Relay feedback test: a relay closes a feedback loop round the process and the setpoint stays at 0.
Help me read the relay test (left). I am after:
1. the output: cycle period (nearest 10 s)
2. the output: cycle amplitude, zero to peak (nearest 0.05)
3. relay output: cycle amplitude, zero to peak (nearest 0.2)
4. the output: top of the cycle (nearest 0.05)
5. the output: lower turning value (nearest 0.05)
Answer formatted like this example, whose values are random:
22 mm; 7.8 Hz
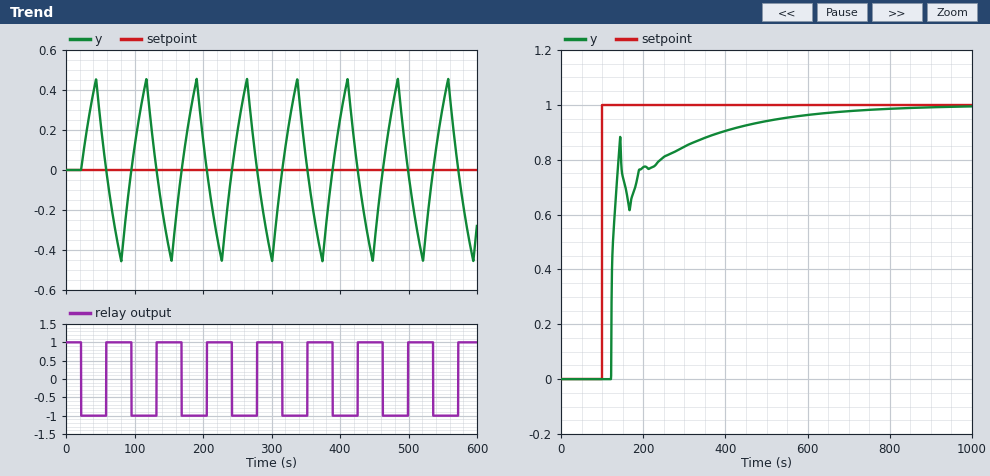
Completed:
70 s; 0.45; 1.0; 0.45; -0.45
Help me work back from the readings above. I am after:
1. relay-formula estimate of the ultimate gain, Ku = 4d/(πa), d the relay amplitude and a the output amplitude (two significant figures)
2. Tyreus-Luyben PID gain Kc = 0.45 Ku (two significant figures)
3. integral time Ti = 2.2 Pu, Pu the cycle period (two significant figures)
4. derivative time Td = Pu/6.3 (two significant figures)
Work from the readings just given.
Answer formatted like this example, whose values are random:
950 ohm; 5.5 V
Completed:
2.8; 1.3; 150 s; 11 s
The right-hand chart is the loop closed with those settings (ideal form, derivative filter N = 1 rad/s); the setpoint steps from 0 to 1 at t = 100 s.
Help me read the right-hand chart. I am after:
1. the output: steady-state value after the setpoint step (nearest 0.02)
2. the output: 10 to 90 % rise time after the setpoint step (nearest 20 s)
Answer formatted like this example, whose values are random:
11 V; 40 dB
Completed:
1.00; 260 s
